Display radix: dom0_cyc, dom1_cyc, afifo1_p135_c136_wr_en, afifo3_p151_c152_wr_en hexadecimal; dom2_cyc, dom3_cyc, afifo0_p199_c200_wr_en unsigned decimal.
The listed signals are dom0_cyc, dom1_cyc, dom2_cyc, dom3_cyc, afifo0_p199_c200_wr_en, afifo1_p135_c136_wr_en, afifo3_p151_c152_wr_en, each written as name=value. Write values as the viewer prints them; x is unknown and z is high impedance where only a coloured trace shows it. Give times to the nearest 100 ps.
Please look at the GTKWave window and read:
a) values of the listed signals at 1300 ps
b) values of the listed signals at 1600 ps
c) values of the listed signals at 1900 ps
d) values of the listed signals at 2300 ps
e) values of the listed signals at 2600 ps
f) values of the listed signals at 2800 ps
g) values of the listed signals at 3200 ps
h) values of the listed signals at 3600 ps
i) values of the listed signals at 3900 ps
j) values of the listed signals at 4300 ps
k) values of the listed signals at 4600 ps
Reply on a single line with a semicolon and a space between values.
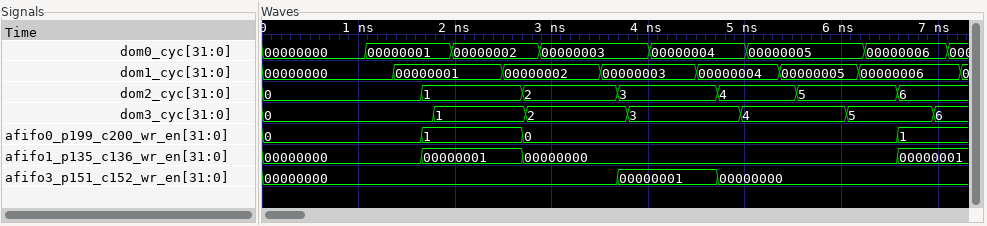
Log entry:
dom0_cyc=00000001, dom1_cyc=00000000, dom2_cyc=0, dom3_cyc=0, afifo0_p199_c200_wr_en=0, afifo1_p135_c136_wr_en=00000000, afifo3_p151_c152_wr_en=00000000; dom0_cyc=00000001, dom1_cyc=00000001, dom2_cyc=0, dom3_cyc=0, afifo0_p199_c200_wr_en=0, afifo1_p135_c136_wr_en=00000000, afifo3_p151_c152_wr_en=00000000; dom0_cyc=00000001, dom1_cyc=00000001, dom2_cyc=1, dom3_cyc=1, afifo0_p199_c200_wr_en=1, afifo1_p135_c136_wr_en=00000001, afifo3_p151_c152_wr_en=00000000; dom0_cyc=00000002, dom1_cyc=00000001, dom2_cyc=1, dom3_cyc=1, afifo0_p199_c200_wr_en=1, afifo1_p135_c136_wr_en=00000001, afifo3_p151_c152_wr_en=00000000; dom0_cyc=00000002, dom1_cyc=00000002, dom2_cyc=1, dom3_cyc=1, afifo0_p199_c200_wr_en=1, afifo1_p135_c136_wr_en=00000001, afifo3_p151_c152_wr_en=00000000; dom0_cyc=00000002, dom1_cyc=00000002, dom2_cyc=2, dom3_cyc=2, afifo0_p199_c200_wr_en=0, afifo1_p135_c136_wr_en=00000000, afifo3_p151_c152_wr_en=00000000; dom0_cyc=00000003, dom1_cyc=00000002, dom2_cyc=2, dom3_cyc=2, afifo0_p199_c200_wr_en=0, afifo1_p135_c136_wr_en=00000000, afifo3_p151_c152_wr_en=00000000; dom0_cyc=00000003, dom1_cyc=00000003, dom2_cyc=2, dom3_cyc=2, afifo0_p199_c200_wr_en=0, afifo1_p135_c136_wr_en=00000000, afifo3_p151_c152_wr_en=00000000; dom0_cyc=00000003, dom1_cyc=00000003, dom2_cyc=3, dom3_cyc=3, afifo0_p199_c200_wr_en=0, afifo1_p135_c136_wr_en=00000000, afifo3_p151_c152_wr_en=00000001; dom0_cyc=00000004, dom1_cyc=00000003, dom2_cyc=3, dom3_cyc=3, afifo0_p199_c200_wr_en=0, afifo1_p135_c136_wr_en=00000000, afifo3_p151_c152_wr_en=00000001; dom0_cyc=00000004, dom1_cyc=00000004, dom2_cyc=3, dom3_cyc=3, afifo0_p199_c200_wr_en=0, afifo1_p135_c136_wr_en=00000000, afifo3_p151_c152_wr_en=00000001
